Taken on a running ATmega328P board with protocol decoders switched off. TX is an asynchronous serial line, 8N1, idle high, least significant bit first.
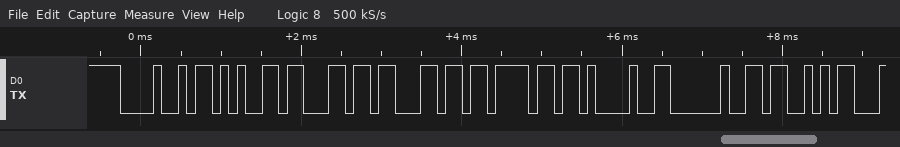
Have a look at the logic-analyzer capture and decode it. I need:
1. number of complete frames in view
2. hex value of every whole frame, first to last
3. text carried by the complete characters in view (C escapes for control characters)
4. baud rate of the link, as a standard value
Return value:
8
0x48 0x65 0x6C 0x6C 0x6F 0x21 0x20 0x53
"Hello! S"
9600 baud
